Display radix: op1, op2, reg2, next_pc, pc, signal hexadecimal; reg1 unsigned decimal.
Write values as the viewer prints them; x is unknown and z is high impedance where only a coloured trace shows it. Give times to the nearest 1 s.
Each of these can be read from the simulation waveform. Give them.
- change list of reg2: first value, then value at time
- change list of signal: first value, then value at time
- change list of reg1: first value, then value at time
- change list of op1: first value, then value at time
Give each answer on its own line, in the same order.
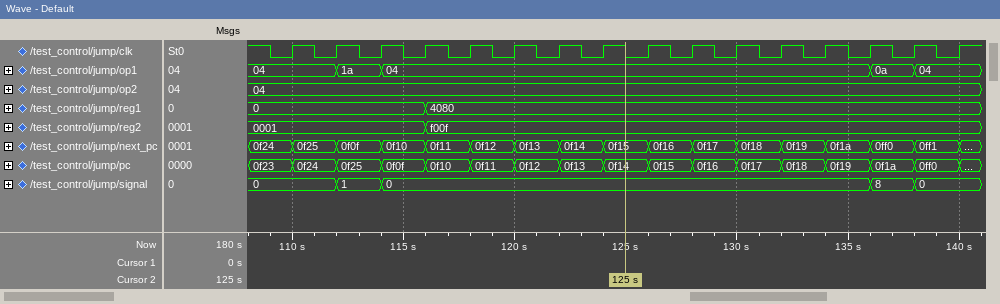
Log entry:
0001, f00f at 116 s
0, 1 at 112 s, 0 at 114 s, 8 at 136 s, 0 at 138 s
0, 4080 at 116 s
04, 1a at 112 s, 04 at 114 s, 0a at 136 s, 04 at 138 s
